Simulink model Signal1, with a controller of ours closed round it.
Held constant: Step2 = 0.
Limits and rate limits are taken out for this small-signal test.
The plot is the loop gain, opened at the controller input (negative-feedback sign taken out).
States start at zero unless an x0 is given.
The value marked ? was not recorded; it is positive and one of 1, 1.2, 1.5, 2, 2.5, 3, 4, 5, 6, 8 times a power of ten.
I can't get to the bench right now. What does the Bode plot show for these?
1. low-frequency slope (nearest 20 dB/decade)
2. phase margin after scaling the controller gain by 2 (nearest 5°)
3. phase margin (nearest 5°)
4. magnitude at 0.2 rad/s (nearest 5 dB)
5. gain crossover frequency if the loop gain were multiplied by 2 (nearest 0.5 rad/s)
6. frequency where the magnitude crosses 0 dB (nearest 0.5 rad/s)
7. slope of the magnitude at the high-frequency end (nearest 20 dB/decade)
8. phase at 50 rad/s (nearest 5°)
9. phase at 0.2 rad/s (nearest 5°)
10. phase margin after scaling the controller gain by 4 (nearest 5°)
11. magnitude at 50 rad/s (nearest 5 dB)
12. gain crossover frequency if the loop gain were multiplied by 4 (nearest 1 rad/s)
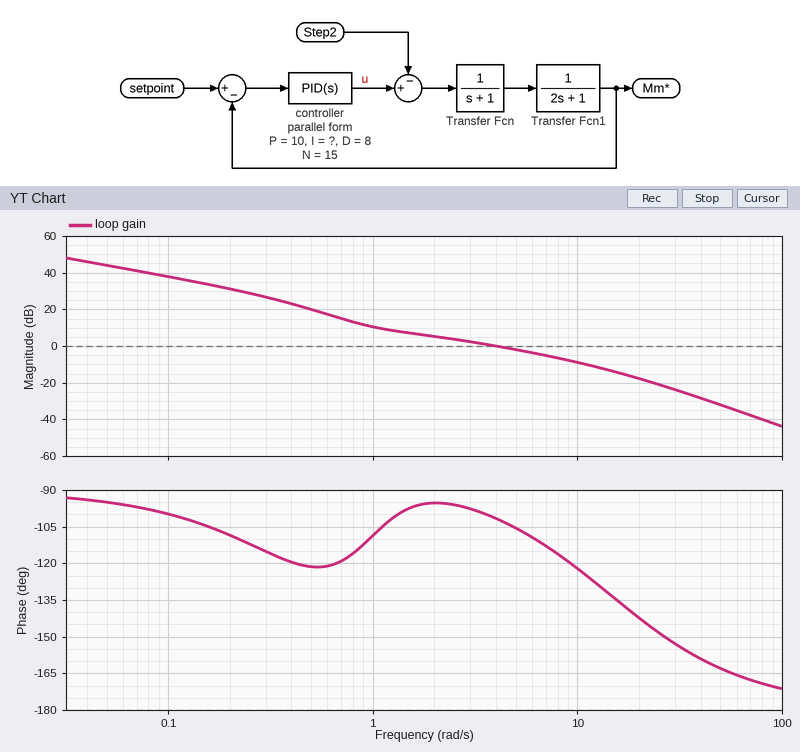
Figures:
-20 dB/decade
65°
80°
30 dB
7.5 rad/s
4.0 rad/s
-40 dB/decade
-165°
-110°
50°
-30 dB
13 rad/s
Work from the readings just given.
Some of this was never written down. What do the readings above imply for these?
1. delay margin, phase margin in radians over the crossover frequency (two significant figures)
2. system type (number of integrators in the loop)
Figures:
0.35 s
1
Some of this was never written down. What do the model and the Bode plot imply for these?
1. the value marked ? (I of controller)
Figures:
8
